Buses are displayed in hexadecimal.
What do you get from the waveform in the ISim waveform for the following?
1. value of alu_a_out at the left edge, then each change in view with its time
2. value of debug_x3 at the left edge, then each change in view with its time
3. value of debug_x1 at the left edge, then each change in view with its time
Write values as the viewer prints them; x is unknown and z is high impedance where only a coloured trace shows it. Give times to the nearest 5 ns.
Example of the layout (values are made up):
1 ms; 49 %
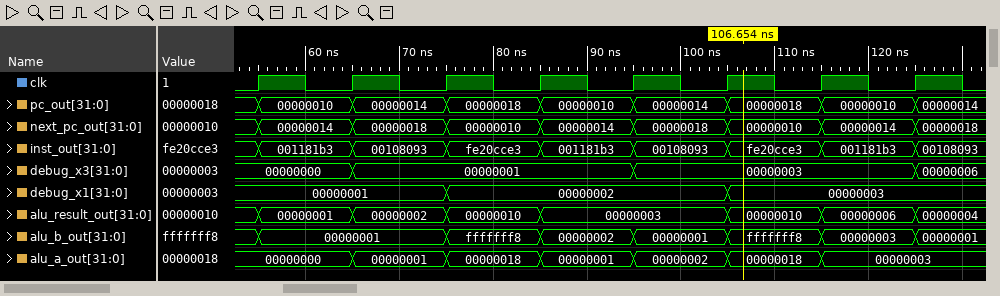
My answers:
00000000, 00000001 at 65 ns, 00000018 at 75 ns, 00000001 at 85 ns, 00000002 at 95 ns, 00000018 at 105 ns, 00000003 at 115 ns; 00000000, 00000001 at 65 ns, 00000003 at 95 ns, 00000006 at 125 ns; 00000001, 00000002 at 75 ns, 00000003 at 105 ns
